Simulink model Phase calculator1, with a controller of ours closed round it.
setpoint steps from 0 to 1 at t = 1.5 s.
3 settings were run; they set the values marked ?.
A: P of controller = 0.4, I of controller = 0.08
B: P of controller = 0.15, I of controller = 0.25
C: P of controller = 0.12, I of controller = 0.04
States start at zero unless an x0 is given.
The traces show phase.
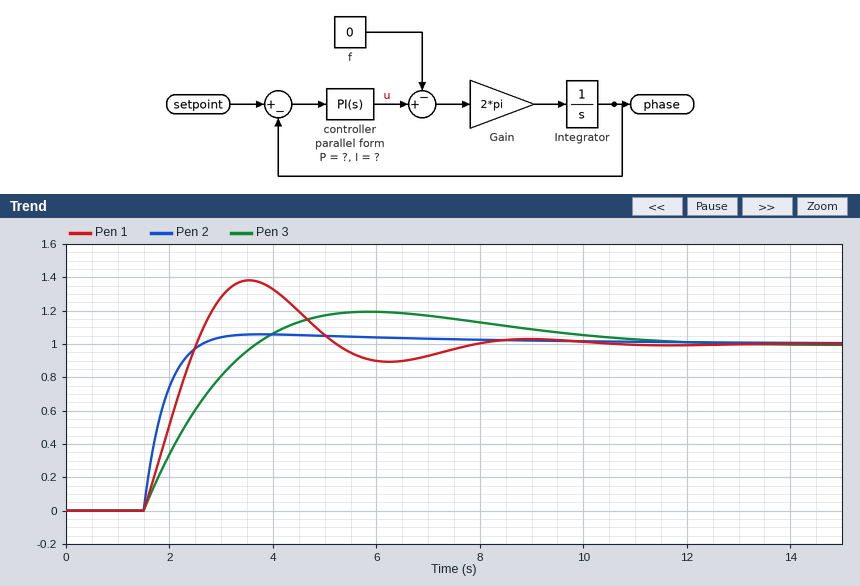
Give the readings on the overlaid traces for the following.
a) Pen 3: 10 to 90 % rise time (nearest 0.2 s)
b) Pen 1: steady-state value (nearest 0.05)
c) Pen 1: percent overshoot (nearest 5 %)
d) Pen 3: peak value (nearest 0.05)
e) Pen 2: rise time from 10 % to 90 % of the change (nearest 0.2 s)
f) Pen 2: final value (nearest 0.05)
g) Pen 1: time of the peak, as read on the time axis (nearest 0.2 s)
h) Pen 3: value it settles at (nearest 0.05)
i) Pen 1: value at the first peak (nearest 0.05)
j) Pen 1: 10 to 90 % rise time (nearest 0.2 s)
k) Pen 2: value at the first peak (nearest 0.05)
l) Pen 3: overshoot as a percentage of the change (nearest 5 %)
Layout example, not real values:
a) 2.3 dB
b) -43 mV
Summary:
a) 1.6 s
b) 1.00
c) 40 %
d) 1.20
e) 0.8 s
f) 1.00
g) 3.6 s
h) 1.00
i) 1.40
j) 0.8 s
k) 1.05
l) 20 %
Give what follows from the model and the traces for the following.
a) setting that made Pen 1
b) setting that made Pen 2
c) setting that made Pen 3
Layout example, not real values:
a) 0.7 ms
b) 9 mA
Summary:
a) B
b) A
c) C
